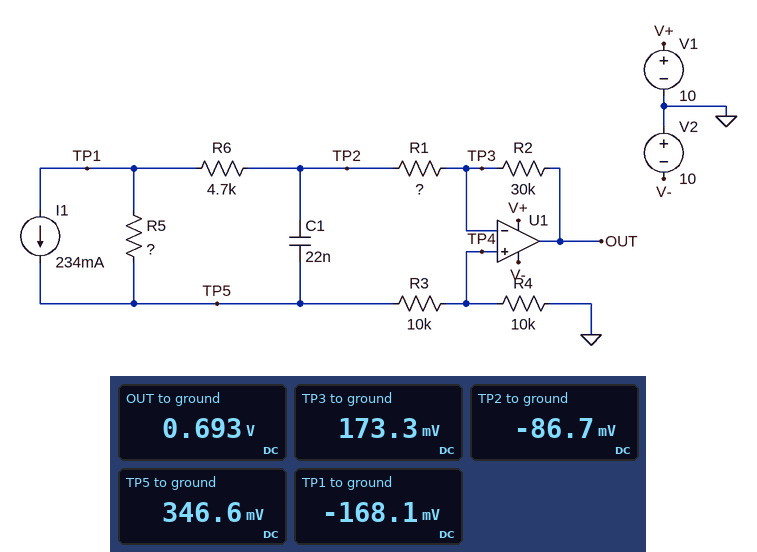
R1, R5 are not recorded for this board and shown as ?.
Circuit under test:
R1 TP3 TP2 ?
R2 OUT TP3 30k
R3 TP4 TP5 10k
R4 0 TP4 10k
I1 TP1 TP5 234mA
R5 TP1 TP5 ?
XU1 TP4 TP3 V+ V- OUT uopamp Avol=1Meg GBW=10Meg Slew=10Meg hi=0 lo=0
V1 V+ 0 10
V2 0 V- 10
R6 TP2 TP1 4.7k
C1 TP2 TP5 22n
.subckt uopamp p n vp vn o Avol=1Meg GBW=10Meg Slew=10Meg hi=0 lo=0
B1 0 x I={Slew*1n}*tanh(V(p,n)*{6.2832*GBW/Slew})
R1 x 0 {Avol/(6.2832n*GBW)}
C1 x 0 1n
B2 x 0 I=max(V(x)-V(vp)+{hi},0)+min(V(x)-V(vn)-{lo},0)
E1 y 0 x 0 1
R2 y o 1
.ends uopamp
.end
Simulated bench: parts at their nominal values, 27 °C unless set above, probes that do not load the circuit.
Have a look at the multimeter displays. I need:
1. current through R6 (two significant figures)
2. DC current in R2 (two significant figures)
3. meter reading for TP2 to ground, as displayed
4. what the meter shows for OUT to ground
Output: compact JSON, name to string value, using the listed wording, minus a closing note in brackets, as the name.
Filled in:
{"current through R6": "17 µA", "DC current in R2": "17 µA", "meter reading for TP2 to ground, as displayed": "-86.7 mV", "what the meter shows for OUT to ground": "0.693 V"}
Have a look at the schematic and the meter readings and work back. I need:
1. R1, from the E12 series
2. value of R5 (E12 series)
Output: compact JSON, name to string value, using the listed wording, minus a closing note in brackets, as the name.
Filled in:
{"R1, from the E12 series": "15 kΩ", "value of R5": "2.2 Ω"}
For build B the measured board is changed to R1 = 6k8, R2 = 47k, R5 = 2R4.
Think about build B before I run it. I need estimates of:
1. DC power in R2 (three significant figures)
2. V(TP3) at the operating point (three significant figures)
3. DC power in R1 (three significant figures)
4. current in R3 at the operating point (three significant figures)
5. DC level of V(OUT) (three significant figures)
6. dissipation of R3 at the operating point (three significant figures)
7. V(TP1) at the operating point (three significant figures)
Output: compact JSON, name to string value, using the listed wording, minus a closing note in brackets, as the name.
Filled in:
{"DC power in R2": "32.1 µW", "V(TP3) at the operating point": "261 mV", "DC power in R1": "4.64 µW", "current in R3 at the operating point": "26.1 µA", "DC level of V(OUT)": "1.49 V", "dissipation of R3 at the operating point": "6.82 µW", "V(TP1) at the operating point": "-39.2 mV"}
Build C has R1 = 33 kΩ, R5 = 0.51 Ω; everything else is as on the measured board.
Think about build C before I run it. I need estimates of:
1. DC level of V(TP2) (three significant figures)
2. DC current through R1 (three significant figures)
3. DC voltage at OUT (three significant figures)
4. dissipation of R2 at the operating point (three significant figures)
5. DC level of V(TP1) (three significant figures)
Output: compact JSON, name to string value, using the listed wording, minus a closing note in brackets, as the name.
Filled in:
{"DC level of V(TP2)": "-57.5 mV", "DC current through R1": "2.50 µA", "DC voltage at OUT": "100 mV", "dissipation of R2 at the operating point": "188 nW", "DC level of V(TP1)": "-69.3 mV"}
